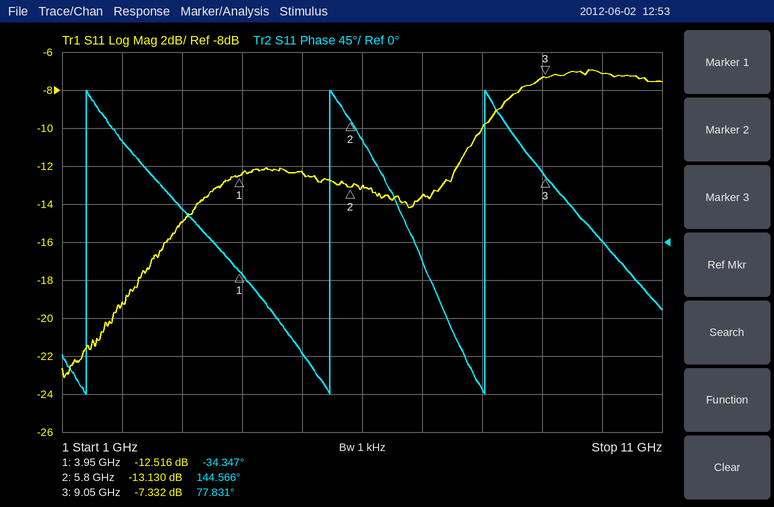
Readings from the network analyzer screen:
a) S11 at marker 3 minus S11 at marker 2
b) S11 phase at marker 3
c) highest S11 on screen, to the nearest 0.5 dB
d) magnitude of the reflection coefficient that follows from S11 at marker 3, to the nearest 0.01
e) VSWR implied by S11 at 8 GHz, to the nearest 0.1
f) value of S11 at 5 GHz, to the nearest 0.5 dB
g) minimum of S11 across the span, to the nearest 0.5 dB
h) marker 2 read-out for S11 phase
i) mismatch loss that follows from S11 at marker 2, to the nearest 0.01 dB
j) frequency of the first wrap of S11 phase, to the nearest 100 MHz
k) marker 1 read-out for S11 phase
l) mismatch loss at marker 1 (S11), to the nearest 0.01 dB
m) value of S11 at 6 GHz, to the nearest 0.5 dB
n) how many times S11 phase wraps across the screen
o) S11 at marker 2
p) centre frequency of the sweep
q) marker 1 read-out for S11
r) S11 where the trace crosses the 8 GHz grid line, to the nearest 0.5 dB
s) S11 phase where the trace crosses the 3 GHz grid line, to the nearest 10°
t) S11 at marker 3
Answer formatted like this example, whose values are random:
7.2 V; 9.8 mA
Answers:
5.798 dB; 77.831°; -7.0 dB; 0.43; 1.9; -12.5 dB; -23.0 dB; 144.566°; 0.22 dB; 1.4 GHz; -34.347°; 0.25 dB; -13.0 dB; 3; -13.130 dB; 6 GHz; -12.516 dB; -10.0 dB; 40°; -7.332 dB
